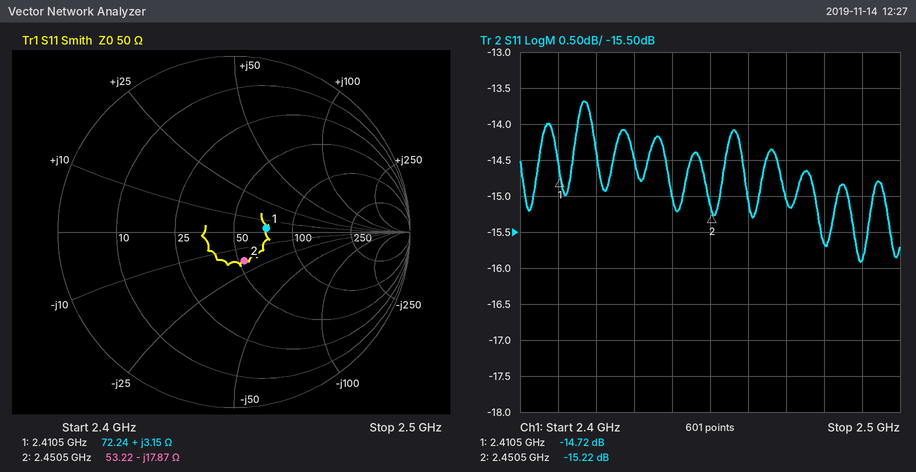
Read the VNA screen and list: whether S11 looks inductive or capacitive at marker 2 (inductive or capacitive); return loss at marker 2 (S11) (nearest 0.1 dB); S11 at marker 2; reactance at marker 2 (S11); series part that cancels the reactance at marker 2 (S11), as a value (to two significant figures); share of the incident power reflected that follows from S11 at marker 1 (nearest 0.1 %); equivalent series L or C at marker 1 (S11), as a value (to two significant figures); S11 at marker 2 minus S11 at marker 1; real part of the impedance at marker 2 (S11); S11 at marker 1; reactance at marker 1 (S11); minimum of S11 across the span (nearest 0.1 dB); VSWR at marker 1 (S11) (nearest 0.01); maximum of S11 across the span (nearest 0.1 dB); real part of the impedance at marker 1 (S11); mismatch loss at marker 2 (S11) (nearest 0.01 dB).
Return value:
capacitive
15.2 dB
-15.22 dB
-17.87 Ω
1.2 nH
3.4 %
210 pH
-0.50 dB
53.22 Ω
-14.72 dB
+3.15 Ω
-15.9 dB
1.45
-13.7 dB
72.24 Ω
0.13 dB
